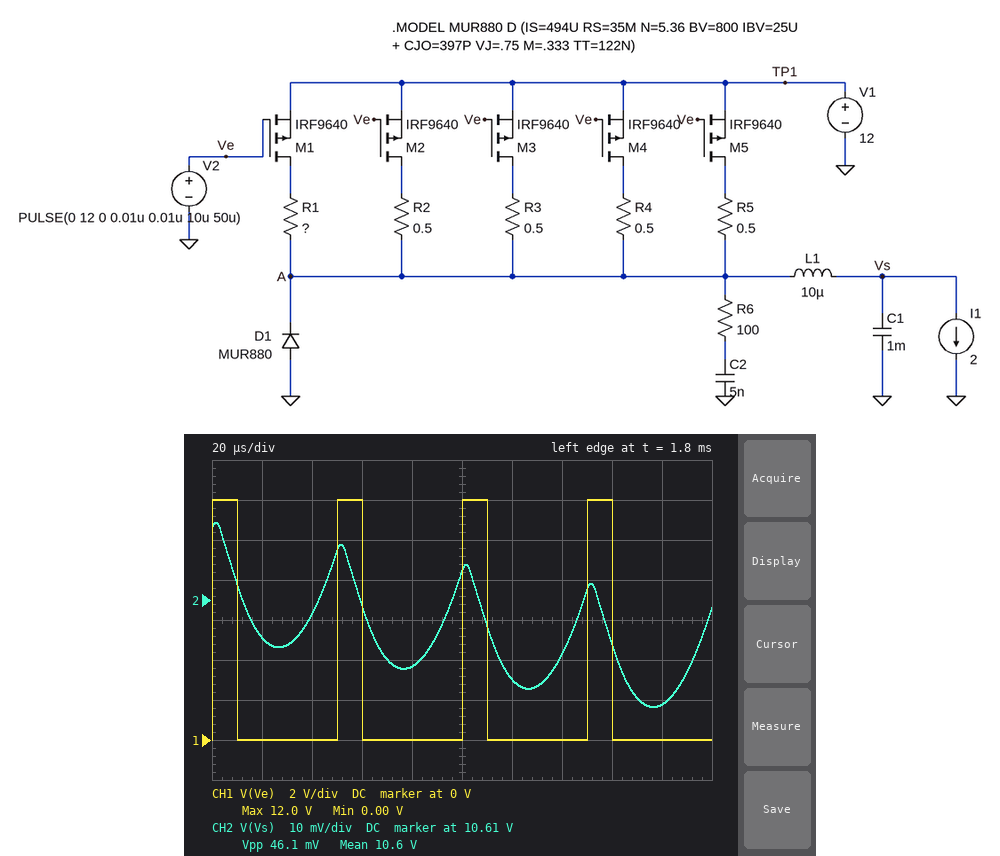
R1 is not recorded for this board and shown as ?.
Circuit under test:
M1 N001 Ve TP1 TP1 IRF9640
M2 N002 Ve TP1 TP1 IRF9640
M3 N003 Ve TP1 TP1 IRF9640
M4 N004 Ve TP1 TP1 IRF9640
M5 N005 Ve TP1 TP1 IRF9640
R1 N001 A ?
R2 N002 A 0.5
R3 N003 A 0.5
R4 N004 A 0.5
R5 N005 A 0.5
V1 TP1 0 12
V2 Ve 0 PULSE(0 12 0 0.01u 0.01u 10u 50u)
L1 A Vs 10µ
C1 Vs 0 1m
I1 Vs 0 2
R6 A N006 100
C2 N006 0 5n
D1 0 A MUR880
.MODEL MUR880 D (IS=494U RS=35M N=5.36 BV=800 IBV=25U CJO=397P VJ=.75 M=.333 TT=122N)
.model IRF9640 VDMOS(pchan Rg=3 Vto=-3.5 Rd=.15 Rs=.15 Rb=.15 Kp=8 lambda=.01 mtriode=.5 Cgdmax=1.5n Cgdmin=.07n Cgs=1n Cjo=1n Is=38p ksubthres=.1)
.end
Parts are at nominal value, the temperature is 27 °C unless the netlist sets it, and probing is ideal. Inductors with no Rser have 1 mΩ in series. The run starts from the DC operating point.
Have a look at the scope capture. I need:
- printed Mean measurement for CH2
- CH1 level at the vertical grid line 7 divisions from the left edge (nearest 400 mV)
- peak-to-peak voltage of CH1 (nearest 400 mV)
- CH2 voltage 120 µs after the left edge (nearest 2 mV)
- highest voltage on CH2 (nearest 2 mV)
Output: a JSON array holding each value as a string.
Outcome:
["10.6 V", "0 V", "12.0 V", "10.590 V", "10.630 V"]
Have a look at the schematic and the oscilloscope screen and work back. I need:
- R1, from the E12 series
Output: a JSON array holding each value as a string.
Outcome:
["1.5 Ω"]
